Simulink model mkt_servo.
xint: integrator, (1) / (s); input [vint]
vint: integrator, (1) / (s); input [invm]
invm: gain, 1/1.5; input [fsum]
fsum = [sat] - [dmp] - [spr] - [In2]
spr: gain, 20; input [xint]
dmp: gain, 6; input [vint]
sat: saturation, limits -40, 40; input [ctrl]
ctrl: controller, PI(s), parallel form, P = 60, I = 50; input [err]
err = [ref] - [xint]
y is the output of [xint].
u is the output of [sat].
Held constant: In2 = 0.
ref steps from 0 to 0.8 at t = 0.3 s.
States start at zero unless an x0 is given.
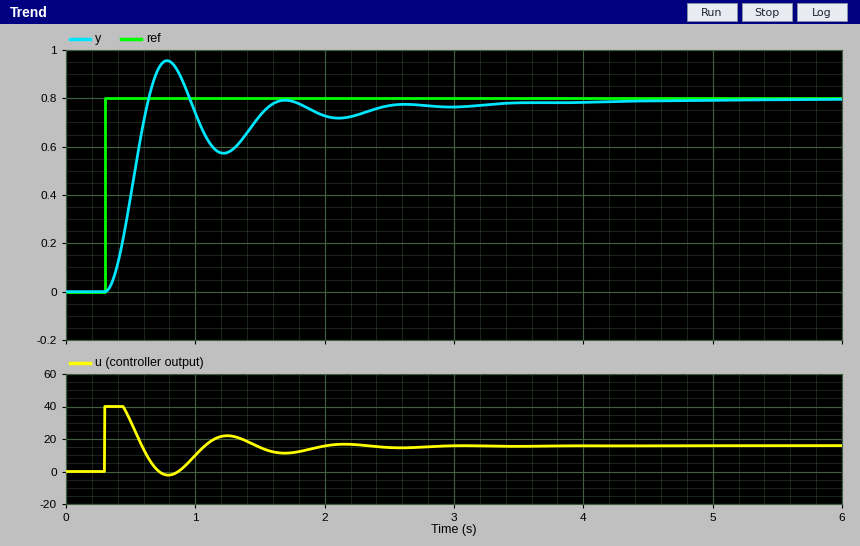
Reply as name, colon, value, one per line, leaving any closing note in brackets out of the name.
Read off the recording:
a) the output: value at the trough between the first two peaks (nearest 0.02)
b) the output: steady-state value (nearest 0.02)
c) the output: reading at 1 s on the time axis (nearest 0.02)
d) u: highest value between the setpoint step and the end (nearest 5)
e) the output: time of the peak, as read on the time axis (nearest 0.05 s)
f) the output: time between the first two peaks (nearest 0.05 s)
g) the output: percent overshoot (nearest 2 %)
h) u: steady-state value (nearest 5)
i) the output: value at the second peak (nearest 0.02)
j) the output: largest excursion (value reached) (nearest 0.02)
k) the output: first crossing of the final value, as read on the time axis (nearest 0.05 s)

the output: value at the trough between the first two peaks: 0.58
the output: steady-state value: 0.80
the output: reading at 1 s on the time axis: 0.74
u: highest value between the setpoint step and the end: 40
the output: time of the peak, as read on the time axis: 0.80 s
the output: time between the first two peaks: 0.90 s
the output: percent overshoot: 20 %
u: steady-state value: 15
the output: value at the second peak: 0.80
the output: largest excursion (value reached): 0.96
the output: first crossing of the final value, as read on the time axis: 0.65 s
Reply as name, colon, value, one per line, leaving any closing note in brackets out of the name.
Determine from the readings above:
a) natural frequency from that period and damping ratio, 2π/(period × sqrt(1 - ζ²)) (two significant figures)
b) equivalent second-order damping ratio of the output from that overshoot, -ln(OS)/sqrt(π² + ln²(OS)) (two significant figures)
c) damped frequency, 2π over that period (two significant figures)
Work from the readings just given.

natural frequency from that period and damping ratio, 2π/(period × sqrt(1 - ζ²)): 7.9 rad/s
equivalent second-order damping ratio of the output from that overshoot, -ln(OS)/sqrt(π² + ln²(OS)): 0.46
damped frequency, 2π over that period: 7.0 rad/s
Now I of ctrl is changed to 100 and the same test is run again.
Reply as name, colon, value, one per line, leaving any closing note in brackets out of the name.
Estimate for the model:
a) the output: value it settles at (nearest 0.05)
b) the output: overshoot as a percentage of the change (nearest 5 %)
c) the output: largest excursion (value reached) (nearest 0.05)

the output: value it settles at: 0.80
the output: overshoot as a percentage of the change: 35 %
the output: largest excursion (value reached): 1.05
